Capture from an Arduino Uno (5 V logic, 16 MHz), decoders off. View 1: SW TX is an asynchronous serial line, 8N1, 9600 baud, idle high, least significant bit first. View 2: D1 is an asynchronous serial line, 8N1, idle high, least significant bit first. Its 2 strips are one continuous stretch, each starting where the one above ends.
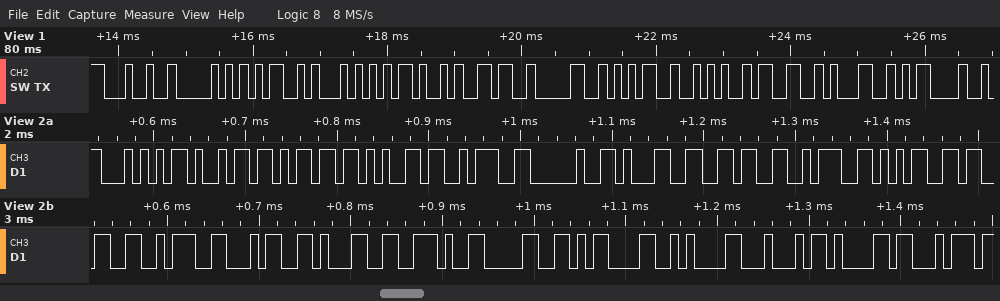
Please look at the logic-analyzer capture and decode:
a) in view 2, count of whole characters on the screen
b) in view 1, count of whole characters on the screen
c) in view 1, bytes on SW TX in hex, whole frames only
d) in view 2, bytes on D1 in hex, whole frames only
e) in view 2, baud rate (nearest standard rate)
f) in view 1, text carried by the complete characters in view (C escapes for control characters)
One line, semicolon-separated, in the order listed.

21; 12; 0x24 0x50 0x4D 0x54 0x4B 0x36 0x30 0x35 0x2A 0x33 0x31 0x0D; 0x54 0x69 0x6D 0x65 0x3A 0x20 0x31 0x36 0x3A 0x35 0x33 0x3A 0x34 0x31 0x2E 0x30 0x0D 0x0A 0x44 0x61 0x74; 115200 baud; "$PMTK605*31\r"
